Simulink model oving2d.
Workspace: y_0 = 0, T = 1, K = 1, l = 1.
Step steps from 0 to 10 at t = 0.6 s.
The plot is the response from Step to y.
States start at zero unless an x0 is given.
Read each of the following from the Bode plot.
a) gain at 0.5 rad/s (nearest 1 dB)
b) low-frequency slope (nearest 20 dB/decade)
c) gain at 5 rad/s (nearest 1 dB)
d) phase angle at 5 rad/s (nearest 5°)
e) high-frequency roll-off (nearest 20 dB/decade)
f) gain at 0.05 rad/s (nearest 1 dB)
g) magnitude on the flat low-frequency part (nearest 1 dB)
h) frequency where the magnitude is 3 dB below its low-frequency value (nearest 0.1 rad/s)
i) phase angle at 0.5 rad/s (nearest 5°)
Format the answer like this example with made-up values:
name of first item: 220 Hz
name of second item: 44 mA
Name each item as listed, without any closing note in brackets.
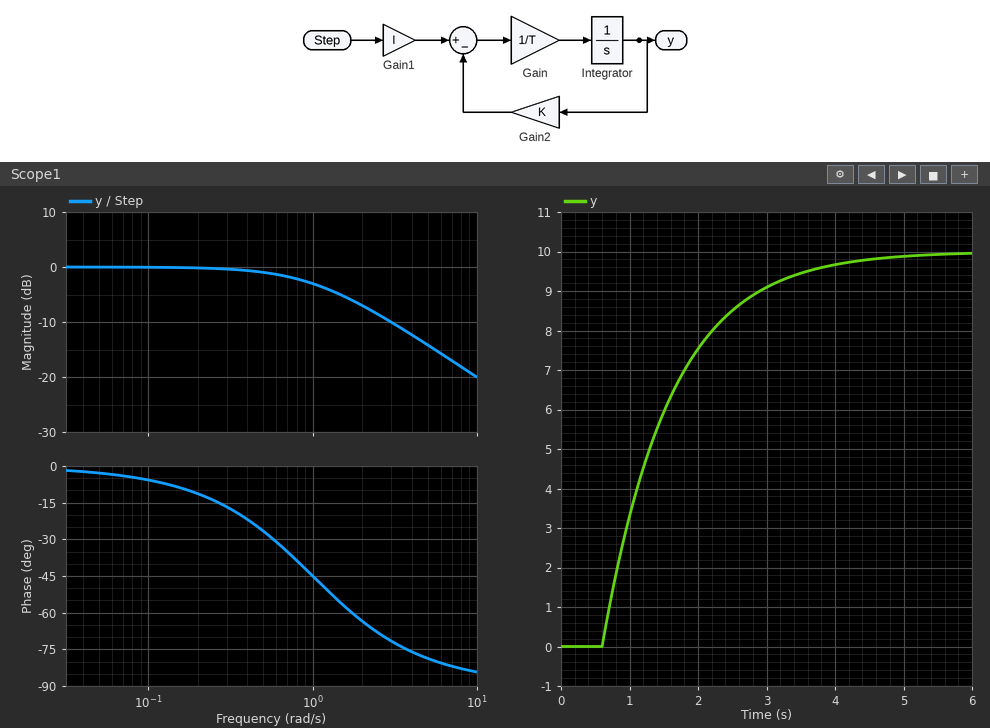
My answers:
gain at 0.5 rad/s: -1 dB
low-frequency slope: 0 dB/decade
gain at 5 rad/s: -14 dB
phase angle at 5 rad/s: -80°
high-frequency roll-off: -20 dB/decade
gain at 0.05 rad/s: 0 dB
magnitude on the flat low-frequency part: 0 dB
frequency where the magnitude is 3 dB below its low-frequency value: 1.0 rad/s
phase angle at 0.5 rad/s: -25°
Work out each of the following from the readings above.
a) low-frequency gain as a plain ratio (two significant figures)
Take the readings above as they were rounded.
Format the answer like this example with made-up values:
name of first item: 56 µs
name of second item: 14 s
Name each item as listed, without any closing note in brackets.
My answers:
low-frequency gain as a plain ratio: 1.0
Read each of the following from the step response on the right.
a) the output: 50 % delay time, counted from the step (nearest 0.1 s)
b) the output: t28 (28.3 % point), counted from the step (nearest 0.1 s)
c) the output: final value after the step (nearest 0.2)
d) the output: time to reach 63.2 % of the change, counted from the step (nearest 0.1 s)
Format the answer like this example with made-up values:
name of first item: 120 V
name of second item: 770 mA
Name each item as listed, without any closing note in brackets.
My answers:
the output: 50 % delay time, counted from the step: 0.7 s
the output: t28 (28.3 % point), counted from the step: 0.3 s
the output: final value after the step: 10.0
the output: time to reach 63.2 % of the change, counted from the step: 1.0 s
